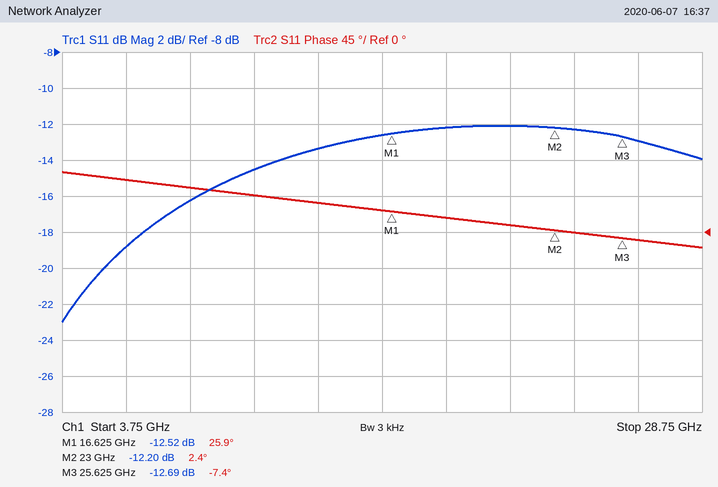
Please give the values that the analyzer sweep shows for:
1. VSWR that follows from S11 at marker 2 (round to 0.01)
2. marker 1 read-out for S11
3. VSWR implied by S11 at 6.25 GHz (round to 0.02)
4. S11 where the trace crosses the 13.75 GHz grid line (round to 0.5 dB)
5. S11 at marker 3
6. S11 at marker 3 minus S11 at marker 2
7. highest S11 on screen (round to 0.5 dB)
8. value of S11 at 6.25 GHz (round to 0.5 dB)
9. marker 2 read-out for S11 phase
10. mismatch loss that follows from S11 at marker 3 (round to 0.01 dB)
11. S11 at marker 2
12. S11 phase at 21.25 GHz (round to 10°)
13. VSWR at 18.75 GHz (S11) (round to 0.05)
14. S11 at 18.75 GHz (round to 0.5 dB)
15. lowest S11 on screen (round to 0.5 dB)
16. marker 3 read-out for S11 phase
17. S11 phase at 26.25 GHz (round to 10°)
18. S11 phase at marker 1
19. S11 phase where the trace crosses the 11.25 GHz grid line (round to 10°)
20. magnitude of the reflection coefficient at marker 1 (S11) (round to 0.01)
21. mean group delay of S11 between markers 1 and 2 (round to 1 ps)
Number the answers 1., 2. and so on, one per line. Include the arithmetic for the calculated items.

1. (1 + 0.2455)/(1 − 0.2455) ≈ 1.65
2. -12.52 dB
3. |Γ| = 10^(-19/20) = 0.1122; VSWR = (1 + 0.1122)/(1 − 0.1122) ≈ 1.25, so 1.26 to the nearest 0.02
4. -13.5 dB
5. -12.69 dB
6. -12.69 − (-12.2) = -0.49 dB
7. -12.0 dB
8. -19.0 dB
9. 2.4°
10. −10 log10(1 − 10^(-12.69/10)) ≈ 0.24 dB
11. -12.20 dB
12. 10°
13. |Γ| = 10^(-12/20) = 0.2512; VSWR = (1 + 0.2512)/(1 − 0.2512) ≈ 1.67, so 1.65 to the nearest 0.05
14. -12.0 dB
15. -23.0 dB
16. -7.4°
17. -10°
18. 25.9°
19. 50°
20. 10^(-12.52/20) ≈ 0.24
21. −(2.4° − (25.9°))/(360° × 6.375 GHz) ≈ 10 ps
